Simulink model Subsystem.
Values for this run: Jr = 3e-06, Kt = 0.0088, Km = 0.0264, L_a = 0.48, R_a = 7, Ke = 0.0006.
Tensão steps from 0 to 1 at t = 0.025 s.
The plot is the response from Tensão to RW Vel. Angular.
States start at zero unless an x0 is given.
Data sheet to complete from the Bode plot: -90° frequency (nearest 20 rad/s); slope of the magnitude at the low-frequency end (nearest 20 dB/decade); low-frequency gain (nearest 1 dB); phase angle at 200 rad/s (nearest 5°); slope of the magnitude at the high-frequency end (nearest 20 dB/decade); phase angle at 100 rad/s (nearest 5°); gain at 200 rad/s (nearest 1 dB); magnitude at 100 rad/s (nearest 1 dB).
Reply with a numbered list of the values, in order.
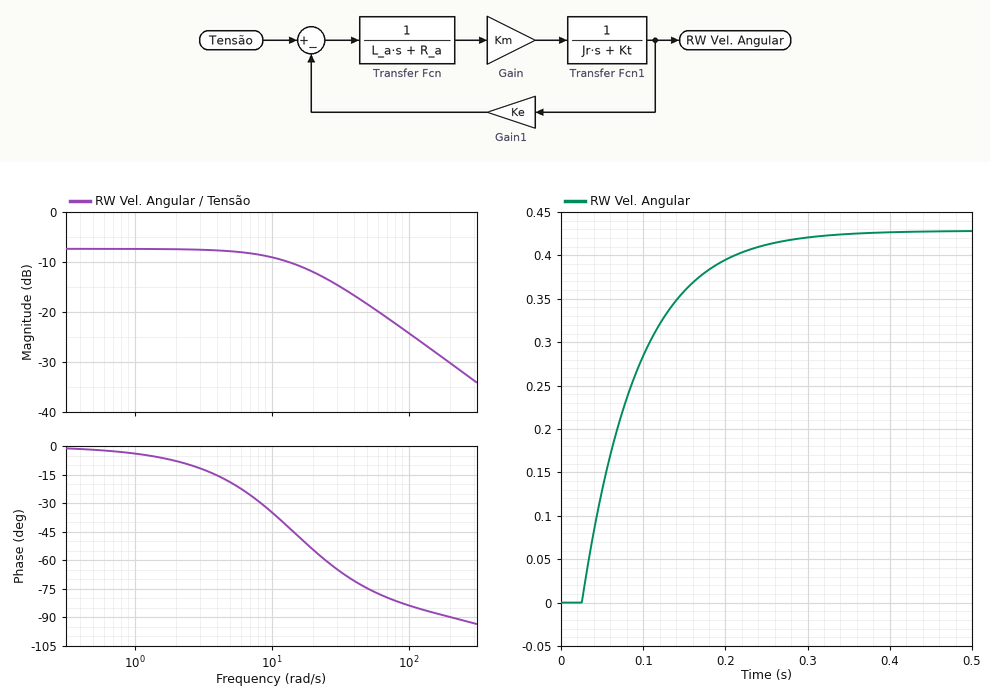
1. 200 rad/s
2. 0 dB/decade
3. -7 dB
4. -90°
5. -20 dB/decade
6. -85°
7. -30 dB
8. -24 dB
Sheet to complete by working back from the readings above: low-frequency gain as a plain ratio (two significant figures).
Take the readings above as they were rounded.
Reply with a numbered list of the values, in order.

1. 0.45
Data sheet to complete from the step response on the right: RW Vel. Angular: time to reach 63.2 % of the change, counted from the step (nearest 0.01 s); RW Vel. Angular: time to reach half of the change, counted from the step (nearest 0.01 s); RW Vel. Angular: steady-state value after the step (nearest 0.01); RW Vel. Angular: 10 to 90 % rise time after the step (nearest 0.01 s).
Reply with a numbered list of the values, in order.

1. 0.07 s
2. 0.05 s
3. 0.43
4. 0.15 s
